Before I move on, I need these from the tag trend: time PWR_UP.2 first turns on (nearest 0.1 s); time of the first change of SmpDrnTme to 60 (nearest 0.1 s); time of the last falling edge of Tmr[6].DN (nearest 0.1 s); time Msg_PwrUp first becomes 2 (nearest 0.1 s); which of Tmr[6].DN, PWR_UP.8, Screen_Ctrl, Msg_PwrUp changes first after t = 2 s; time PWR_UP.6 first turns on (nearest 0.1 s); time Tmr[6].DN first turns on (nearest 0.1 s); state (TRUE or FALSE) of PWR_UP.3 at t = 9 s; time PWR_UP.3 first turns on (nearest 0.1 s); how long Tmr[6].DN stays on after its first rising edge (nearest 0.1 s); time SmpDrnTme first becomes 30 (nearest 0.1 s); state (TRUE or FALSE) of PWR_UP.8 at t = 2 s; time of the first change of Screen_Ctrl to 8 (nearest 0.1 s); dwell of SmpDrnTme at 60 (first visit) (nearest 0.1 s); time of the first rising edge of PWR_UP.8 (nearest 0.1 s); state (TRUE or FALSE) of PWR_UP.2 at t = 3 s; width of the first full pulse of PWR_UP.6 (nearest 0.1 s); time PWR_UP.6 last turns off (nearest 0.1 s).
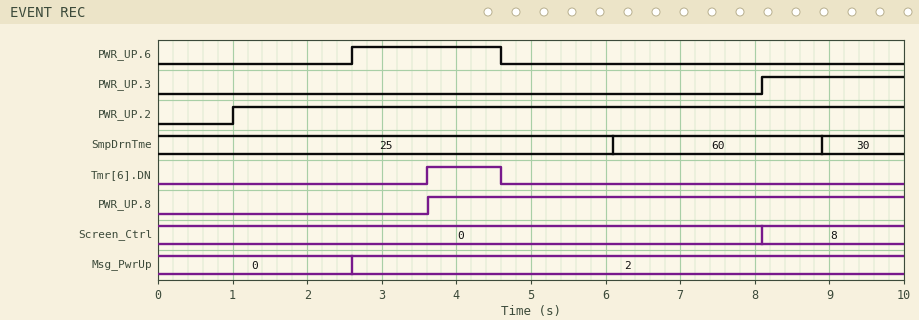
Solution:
1.0 s
6.1 s
4.6 s
2.6 s
Msg_PwrUp
2.6 s
3.6 s
TRUE
8.1 s
1.0 s
8.9 s
FALSE
8.1 s
2.8 s
3.6 s
TRUE
2.0 s
4.6 s
